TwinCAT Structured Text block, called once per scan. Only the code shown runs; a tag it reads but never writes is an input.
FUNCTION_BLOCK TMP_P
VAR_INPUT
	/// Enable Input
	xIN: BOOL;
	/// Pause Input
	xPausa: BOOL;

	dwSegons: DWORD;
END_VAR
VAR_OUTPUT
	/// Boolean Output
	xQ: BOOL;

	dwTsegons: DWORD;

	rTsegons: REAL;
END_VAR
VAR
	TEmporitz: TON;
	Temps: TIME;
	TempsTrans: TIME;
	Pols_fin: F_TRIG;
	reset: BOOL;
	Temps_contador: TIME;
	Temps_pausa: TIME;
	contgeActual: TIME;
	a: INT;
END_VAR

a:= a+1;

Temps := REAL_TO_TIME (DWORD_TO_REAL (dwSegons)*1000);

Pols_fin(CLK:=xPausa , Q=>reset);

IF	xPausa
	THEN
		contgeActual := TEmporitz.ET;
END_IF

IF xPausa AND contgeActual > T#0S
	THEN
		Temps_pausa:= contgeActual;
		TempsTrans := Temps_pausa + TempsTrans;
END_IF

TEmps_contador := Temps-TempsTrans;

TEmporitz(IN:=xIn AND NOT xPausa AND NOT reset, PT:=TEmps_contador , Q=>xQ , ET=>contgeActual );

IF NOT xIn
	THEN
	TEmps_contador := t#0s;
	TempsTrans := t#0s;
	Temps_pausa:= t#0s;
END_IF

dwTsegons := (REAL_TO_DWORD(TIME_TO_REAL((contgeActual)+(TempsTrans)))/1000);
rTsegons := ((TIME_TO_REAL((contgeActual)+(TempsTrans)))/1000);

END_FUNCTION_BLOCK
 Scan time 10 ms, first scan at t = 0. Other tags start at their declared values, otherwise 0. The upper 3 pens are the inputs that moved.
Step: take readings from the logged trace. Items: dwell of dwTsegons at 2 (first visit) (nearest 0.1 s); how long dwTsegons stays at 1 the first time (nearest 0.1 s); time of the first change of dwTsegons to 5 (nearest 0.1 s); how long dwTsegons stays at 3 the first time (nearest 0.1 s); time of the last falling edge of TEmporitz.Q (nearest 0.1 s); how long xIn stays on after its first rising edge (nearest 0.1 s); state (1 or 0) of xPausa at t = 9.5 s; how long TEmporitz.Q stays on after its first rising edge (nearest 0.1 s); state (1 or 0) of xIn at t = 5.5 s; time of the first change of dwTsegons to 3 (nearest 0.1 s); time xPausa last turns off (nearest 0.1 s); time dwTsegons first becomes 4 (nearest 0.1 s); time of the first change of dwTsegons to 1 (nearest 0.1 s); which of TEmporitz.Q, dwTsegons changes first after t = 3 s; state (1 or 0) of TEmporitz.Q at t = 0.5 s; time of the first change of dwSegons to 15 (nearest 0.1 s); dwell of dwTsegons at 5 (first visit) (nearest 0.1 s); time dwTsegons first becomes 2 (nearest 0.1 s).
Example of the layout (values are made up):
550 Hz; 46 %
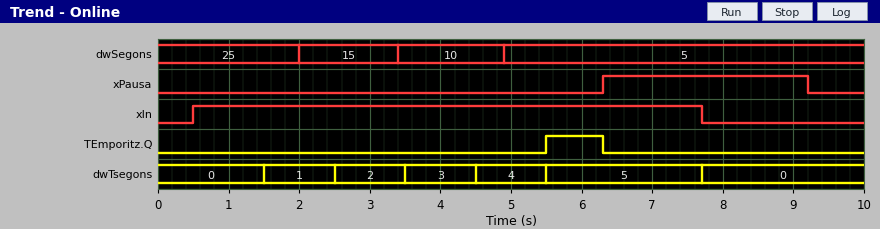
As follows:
1.0 s; 1.0 s; 5.5 s; 1.0 s; 6.3 s; 7.2 s; 0; 0.8 s; 1; 3.5 s; 9.2 s; 4.5 s; 1.5 s; dwTsegons; 0; 2.0 s; 2.2 s; 2.5 s
